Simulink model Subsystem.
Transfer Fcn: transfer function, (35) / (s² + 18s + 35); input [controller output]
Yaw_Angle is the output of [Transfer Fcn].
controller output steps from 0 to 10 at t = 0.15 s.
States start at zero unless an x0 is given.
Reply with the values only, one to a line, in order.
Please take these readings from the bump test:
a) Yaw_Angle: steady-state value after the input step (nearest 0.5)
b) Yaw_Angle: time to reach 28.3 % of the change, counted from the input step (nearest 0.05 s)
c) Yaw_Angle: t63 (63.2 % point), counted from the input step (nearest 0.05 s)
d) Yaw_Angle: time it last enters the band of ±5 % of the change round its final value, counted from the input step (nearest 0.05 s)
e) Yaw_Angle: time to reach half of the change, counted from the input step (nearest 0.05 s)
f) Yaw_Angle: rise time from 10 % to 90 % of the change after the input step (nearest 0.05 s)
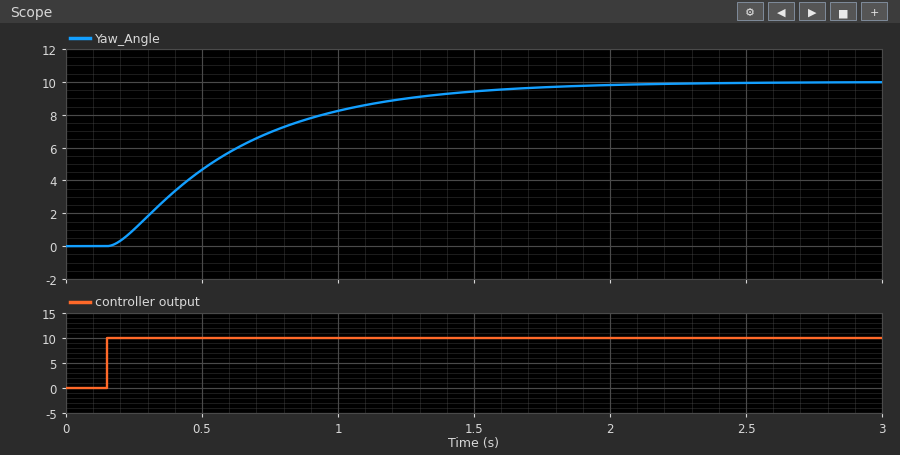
10.0
0.20 s
0.50 s
1.40 s
0.40 s
1.00 s
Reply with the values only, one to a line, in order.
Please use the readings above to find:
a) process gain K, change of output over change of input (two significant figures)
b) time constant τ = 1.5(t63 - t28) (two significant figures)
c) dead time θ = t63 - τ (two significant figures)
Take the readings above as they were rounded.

1.0
0.45 s
0.050 s
